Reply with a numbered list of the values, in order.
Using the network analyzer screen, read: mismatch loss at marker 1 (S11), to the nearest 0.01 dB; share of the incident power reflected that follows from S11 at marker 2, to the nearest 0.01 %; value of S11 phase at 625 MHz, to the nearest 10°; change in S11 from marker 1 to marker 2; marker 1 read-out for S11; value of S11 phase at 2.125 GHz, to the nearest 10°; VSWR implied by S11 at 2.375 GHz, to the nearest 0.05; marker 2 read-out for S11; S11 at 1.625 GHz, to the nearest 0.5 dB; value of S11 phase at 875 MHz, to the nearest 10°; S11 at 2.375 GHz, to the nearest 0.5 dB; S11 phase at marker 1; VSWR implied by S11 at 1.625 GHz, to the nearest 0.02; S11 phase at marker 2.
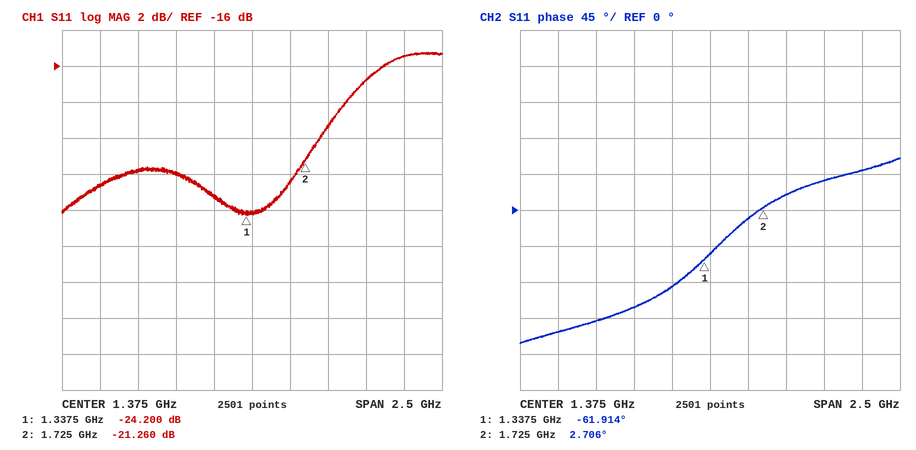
1. 0.02 dB
2. 0.75 %
3. -140°
4. 2.940 dB
5. -24.200 dB
6. 40°
7. 1.40
8. -21.260 dB
9. -22.5 dB
10. -120°
11. -15.5 dB
12. -61.914°
13. 1.16
14. 2.706°
